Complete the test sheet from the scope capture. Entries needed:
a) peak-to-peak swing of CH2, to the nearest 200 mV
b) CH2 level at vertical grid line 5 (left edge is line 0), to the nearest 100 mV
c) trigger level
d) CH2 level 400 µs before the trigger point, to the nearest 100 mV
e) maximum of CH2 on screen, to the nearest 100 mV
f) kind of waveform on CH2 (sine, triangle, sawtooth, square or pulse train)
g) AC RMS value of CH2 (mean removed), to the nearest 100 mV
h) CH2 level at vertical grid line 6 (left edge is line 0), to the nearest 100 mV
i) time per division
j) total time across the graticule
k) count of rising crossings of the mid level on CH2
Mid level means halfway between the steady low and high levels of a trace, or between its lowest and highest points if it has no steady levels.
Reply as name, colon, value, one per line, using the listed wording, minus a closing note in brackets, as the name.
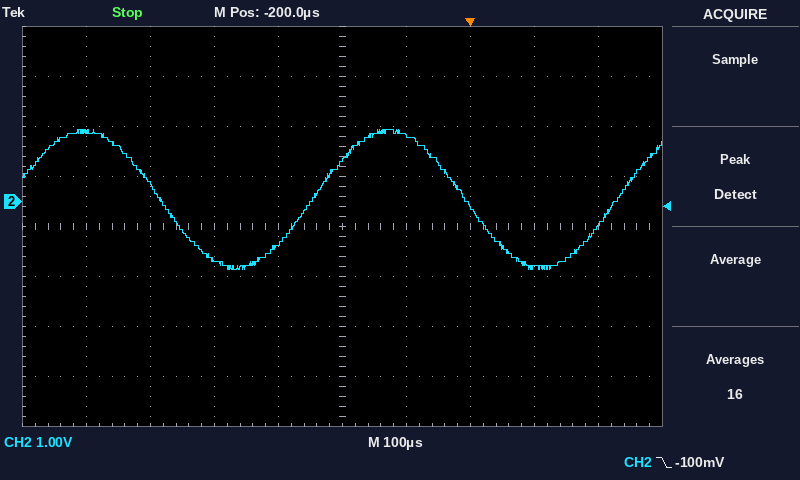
peak-to-peak swing of CH2, to the nearest 200 mV: 2.8 V
CH2 level at vertical grid line 5 (left edge is line 0), to the nearest 100 mV: 800 mV
trigger level: -100 mV
CH2 level 400 µs before the trigger point, to the nearest 100 mV: -1.2 V
maximum of CH2 on screen, to the nearest 100 mV: 1.4 V
kind of waveform on CH2: sine
AC RMS value of CH2 (mean removed), to the nearest 100 mV: 1.0 V
CH2 level at vertical grid line 6 (left edge is line 0), to the nearest 100 mV: 1.3 V
time per division: 100 µs
total time across the graticule: 1 ms
count of rising crossings of the mid level on CH2: 2
